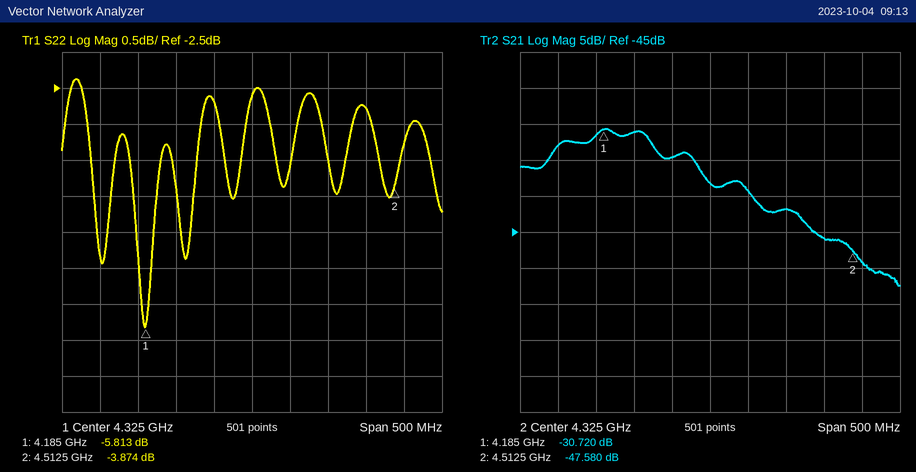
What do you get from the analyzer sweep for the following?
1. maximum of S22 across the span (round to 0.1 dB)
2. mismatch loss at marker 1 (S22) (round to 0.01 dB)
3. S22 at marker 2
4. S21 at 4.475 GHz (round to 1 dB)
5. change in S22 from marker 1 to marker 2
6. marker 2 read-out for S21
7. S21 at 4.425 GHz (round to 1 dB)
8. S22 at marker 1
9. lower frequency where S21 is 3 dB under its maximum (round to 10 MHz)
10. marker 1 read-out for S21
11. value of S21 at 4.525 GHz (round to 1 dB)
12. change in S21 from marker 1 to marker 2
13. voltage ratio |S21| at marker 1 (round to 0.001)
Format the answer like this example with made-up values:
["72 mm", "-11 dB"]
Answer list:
["-2.4 dB", "1.32 dB", "-3.874 dB", "-46 dB", "1.939 dB", "-47.580 dB", "-42 dB", "-5.813 dB", "4.12 GHz", "-30.720 dB", "-49 dB", "-16.860 dB", "0.029"]
